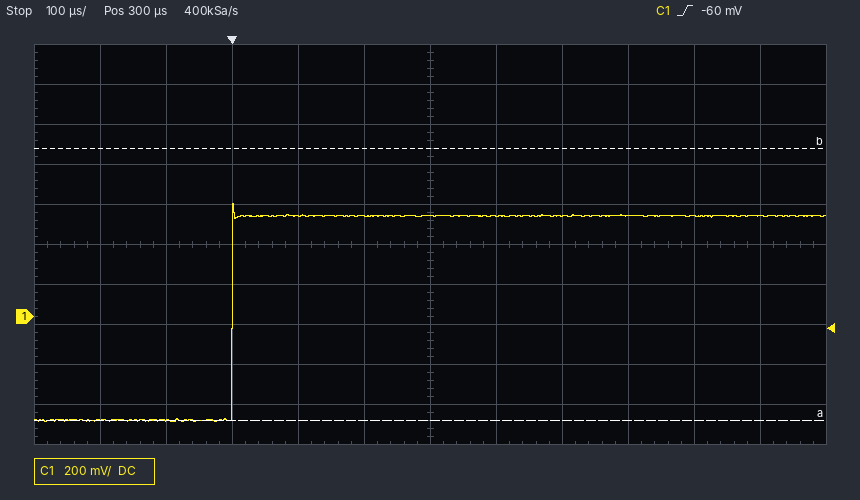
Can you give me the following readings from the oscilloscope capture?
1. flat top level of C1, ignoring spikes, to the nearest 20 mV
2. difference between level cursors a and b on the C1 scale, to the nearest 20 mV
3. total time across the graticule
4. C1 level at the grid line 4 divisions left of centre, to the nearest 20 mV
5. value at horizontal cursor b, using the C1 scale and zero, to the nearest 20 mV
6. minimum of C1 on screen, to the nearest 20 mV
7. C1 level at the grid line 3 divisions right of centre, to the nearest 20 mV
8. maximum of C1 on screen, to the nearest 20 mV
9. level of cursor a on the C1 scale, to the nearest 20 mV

500 mV
1.36 V
1.2 ms
-520 mV
840 mV
-520 mV
500 mV
560 mV
-520 mV
